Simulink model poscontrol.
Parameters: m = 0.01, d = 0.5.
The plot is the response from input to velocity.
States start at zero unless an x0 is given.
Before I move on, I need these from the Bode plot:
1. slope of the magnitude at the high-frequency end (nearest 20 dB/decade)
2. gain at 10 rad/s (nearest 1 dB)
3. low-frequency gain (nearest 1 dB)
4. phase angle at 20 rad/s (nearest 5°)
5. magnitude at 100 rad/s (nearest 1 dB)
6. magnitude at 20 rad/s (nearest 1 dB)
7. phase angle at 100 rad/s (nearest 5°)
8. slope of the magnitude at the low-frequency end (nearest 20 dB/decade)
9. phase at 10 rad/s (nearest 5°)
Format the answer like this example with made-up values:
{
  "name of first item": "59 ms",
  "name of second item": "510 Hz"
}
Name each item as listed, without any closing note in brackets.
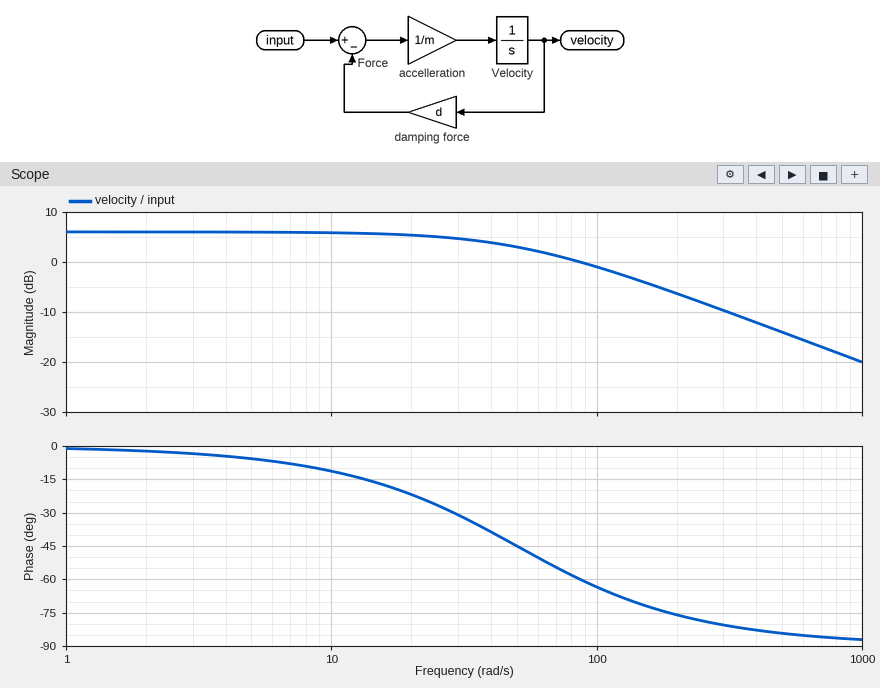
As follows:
{
  "slope of the magnitude at the high-frequency end": "-20 dB/decade",
  "gain at 10 rad/s": "6 dB",
  "low-frequency gain": "6 dB",
  "phase angle at 20 rad/s": "-20°",
  "magnitude at 100 rad/s": "-1 dB",
  "magnitude at 20 rad/s": "5 dB",
  "phase angle at 100 rad/s": "-65°",
  "slope of the magnitude at the low-frequency end": "0 dB/decade",
  "phase at 10 rad/s": "-10°"
}
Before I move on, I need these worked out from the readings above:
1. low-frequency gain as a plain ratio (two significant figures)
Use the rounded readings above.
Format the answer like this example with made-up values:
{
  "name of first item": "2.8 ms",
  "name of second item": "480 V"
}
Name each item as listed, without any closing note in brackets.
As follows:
{
  "low-frequency gain as a plain ratio": "2.0"
}
